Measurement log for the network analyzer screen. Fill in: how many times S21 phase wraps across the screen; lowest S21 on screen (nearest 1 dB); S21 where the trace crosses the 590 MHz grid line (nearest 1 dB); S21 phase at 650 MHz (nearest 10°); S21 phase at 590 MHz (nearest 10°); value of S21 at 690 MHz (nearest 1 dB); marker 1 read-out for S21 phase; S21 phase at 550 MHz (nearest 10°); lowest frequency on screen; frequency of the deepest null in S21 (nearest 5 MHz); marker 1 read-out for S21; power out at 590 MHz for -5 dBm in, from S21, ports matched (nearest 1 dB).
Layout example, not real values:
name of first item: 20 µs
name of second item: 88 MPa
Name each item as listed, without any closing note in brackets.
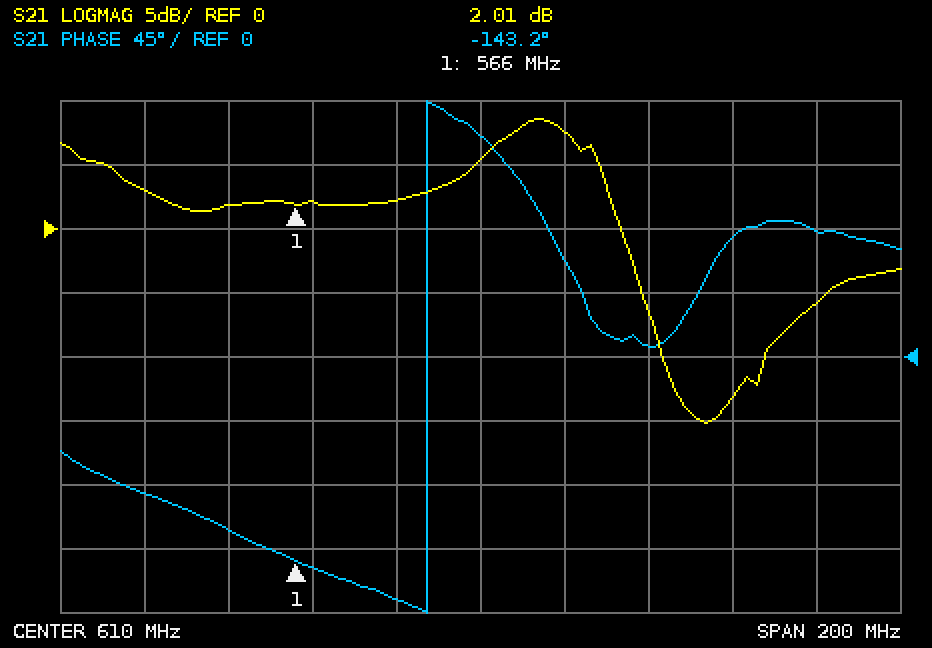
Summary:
how many times S21 phase wraps across the screen: 1
lowest S21 on screen: -15 dB
S21 where the trace crosses the 590 MHz grid line: 2 dB
S21 phase at 650 MHz: 10°
S21 phase at 590 MHz: -170°
value of S21 at 690 MHz: -6 dB
marker 1 read-out for S21 phase: -143.2°
S21 phase at 550 MHz: -120°
lowest frequency on screen: 510 MHz
frequency of the deepest null in S21: 665 MHz
marker 1 read-out for S21: 2.01 dB
power out at 590 MHz for -5 dBm in, from S21, ports matched: -3 dBm
